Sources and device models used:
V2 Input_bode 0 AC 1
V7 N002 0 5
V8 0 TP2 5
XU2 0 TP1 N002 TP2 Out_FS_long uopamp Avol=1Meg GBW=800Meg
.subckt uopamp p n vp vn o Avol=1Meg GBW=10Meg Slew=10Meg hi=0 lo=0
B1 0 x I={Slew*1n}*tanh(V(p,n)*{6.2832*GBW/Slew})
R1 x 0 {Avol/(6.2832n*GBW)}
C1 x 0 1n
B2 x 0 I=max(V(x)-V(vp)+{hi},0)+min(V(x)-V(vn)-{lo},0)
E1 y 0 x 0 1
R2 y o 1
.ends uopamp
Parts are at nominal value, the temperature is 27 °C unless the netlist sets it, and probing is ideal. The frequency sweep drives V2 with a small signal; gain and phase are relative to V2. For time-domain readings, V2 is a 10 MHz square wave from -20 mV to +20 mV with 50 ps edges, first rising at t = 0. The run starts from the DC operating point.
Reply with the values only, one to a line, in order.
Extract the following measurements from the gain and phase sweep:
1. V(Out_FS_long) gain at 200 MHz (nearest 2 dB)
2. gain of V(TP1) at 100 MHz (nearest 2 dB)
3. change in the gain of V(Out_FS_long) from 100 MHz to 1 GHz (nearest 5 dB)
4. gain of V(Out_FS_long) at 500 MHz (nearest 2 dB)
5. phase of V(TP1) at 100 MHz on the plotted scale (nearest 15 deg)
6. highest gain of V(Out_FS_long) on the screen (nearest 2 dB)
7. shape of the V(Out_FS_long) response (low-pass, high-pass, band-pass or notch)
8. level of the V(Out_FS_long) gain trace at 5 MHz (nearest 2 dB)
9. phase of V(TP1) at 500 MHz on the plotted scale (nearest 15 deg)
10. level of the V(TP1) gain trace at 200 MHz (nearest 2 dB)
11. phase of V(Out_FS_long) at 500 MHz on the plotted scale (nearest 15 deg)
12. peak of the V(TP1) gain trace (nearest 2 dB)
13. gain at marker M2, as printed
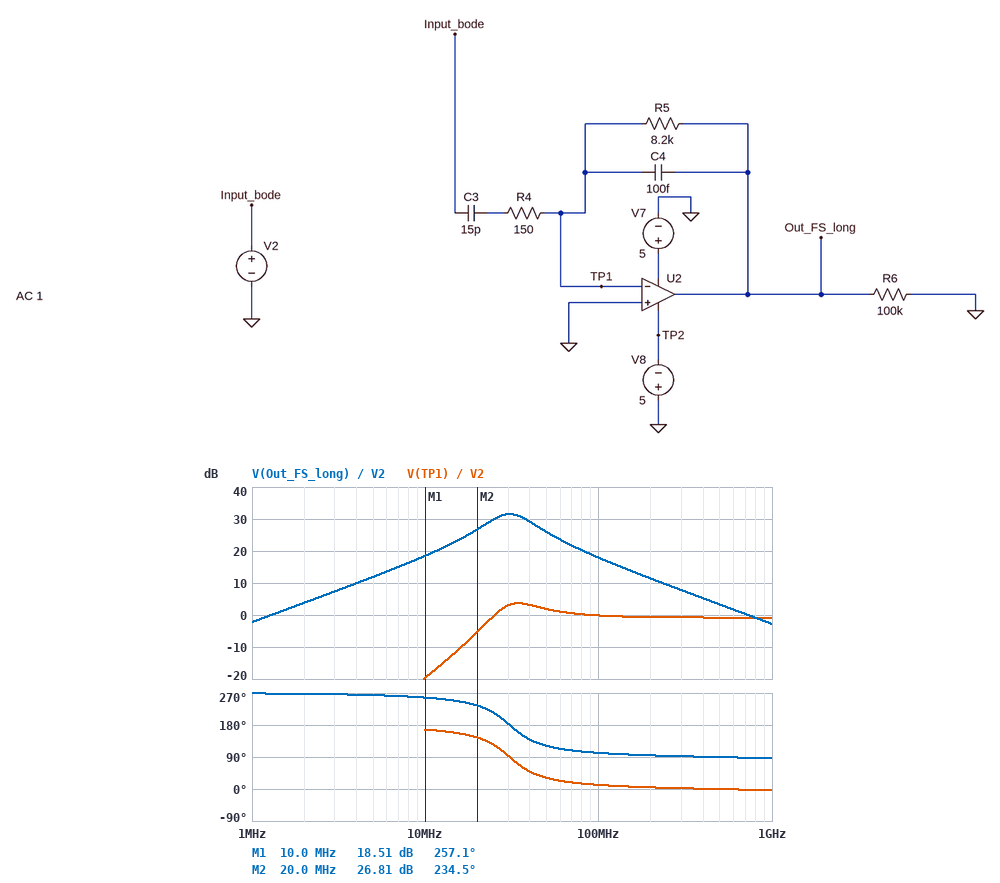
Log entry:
12 dB
0 dB
-20 dB
4 dB
15 deg
32 dB
band-pass
12 dB
0 deg
0 dB
90 deg
4 dB
26.81 dB
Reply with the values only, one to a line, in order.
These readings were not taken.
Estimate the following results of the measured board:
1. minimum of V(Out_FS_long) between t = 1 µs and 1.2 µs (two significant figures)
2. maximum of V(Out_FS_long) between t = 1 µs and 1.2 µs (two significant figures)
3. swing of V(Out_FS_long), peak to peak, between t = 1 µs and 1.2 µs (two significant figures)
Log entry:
-250 mV
250 mV
500 mV
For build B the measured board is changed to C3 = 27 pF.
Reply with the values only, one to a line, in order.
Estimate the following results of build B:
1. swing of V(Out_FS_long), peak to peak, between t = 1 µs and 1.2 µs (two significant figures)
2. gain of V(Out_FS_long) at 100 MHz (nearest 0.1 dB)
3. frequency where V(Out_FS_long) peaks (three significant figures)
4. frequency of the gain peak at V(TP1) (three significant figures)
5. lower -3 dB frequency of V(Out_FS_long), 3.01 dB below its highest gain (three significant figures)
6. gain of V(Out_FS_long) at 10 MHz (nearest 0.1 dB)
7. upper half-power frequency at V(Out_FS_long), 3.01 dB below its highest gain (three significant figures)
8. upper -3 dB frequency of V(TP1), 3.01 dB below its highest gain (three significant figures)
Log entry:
500 mV
17.6 dB
22.9 MHz
26.7 MHz
16.0 MHz
24.1 dB
32.7 MHz
95.5 MHz
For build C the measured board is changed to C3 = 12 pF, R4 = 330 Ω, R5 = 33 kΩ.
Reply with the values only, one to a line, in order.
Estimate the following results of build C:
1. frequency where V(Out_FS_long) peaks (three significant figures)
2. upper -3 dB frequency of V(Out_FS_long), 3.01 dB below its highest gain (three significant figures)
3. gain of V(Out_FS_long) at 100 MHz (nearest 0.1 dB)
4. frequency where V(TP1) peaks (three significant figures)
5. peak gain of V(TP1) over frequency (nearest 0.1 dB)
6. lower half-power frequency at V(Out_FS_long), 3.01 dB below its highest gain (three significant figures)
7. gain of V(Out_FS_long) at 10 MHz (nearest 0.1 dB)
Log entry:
16.5 MHz
24.0 MHz
16.8 dB
19.7 MHz
1.5 dB
11.3 MHz
30.0 dB
